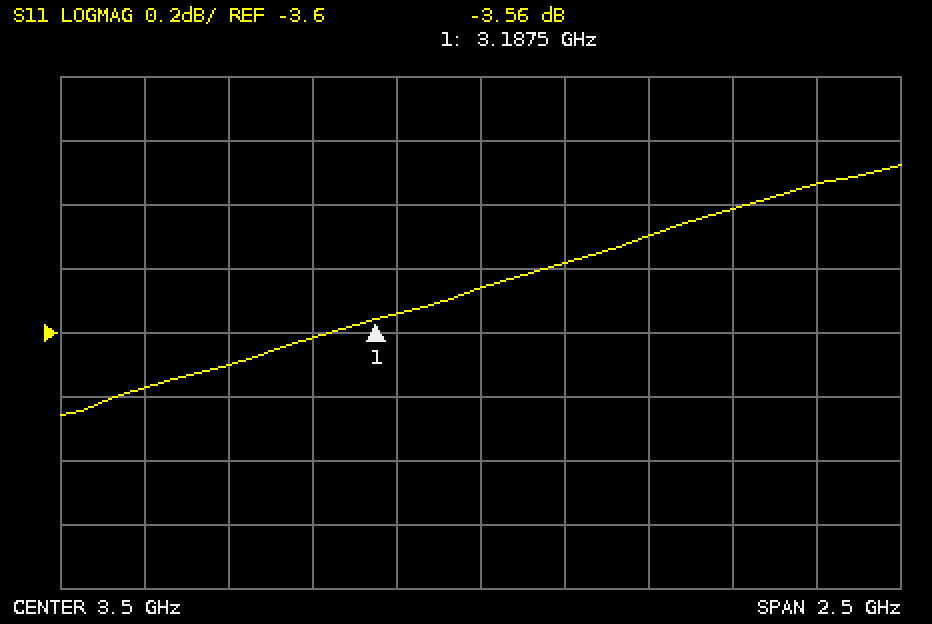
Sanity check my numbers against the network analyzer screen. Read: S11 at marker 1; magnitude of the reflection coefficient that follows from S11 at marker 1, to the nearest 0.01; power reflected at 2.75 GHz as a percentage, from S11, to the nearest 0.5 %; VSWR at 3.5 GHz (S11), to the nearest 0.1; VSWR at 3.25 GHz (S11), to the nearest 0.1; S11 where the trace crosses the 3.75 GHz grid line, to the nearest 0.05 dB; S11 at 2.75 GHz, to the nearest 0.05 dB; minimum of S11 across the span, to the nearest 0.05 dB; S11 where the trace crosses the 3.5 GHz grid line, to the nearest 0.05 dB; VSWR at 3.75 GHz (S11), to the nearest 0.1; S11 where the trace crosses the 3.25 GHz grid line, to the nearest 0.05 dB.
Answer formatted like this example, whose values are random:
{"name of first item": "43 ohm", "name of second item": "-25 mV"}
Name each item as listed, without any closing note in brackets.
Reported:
{"S11 at marker 1": "-3.56 dB", "magnitude of the reflection coefficient that follows from S11 at marker 1, to the nearest 0.01": "0.66", "power reflected at 2.75 GHz as a percentage, from S11, to the nearest 0.5 %": "42.5 %", "VSWR at 3.5 GHz (S11), to the nearest 0.1": "5.1", "VSWR at 3.25 GHz (S11), to the nearest 0.1": "5.0", "S11 where the trace crosses the 3.75 GHz grid line, to the nearest 0.05 dB": "-3.40 dB", "S11 at 2.75 GHz, to the nearest 0.05 dB": "-3.70 dB", "minimum of S11 across the span, to the nearest 0.05 dB": "-3.85 dB", "S11 where the trace crosses the 3.5 GHz grid line, to the nearest 0.05 dB": "-3.45 dB", "VSWR at 3.75 GHz (S11), to the nearest 0.1": "5.2", "S11 where the trace crosses the 3.25 GHz grid line, to the nearest 0.05 dB": "-3.55 dB"}
